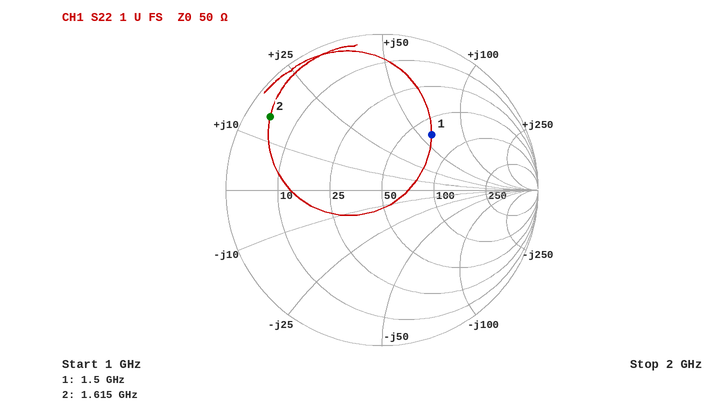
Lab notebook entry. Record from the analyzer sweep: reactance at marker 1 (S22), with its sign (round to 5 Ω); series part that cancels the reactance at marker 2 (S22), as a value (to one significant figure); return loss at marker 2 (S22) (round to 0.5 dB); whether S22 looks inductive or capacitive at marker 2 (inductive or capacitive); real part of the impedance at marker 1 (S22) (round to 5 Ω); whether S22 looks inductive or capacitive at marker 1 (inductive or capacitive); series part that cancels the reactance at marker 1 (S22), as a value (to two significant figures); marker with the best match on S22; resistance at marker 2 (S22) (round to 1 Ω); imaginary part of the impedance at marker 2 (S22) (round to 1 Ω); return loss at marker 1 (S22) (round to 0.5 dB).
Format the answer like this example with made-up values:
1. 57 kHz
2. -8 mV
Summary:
1. +60 Ω
2. 7 pF
3. 1.5 dB
4. inductive
5. 65 Ω
6. inductive
7. 1.8 pF
8. marker 1
9. 4 Ω
10. +15 Ω
11. 6.5 dB
